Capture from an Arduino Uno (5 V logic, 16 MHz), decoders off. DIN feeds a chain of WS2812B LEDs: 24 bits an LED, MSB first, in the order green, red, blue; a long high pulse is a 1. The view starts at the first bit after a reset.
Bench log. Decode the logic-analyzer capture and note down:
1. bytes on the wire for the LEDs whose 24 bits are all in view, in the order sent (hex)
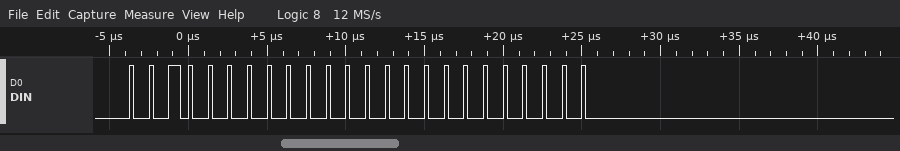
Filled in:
20 00 00
